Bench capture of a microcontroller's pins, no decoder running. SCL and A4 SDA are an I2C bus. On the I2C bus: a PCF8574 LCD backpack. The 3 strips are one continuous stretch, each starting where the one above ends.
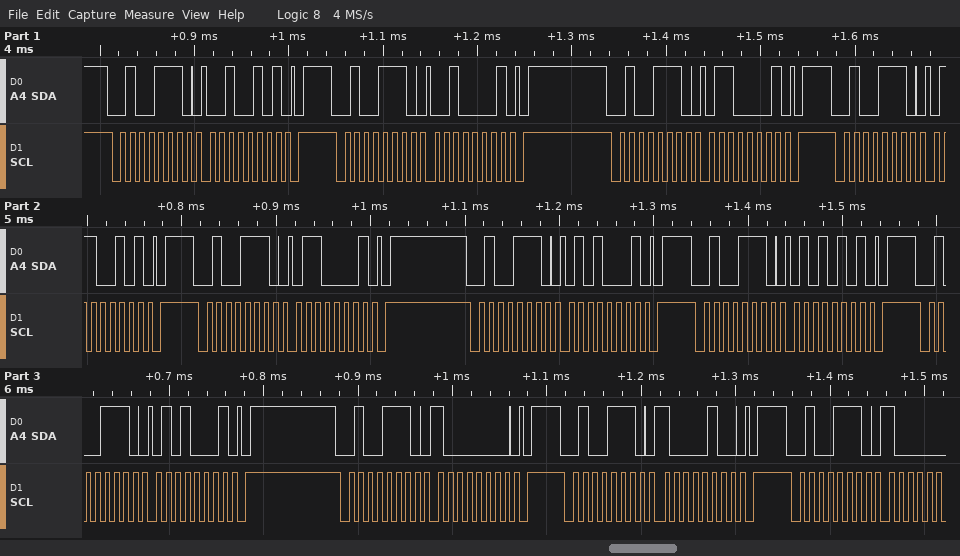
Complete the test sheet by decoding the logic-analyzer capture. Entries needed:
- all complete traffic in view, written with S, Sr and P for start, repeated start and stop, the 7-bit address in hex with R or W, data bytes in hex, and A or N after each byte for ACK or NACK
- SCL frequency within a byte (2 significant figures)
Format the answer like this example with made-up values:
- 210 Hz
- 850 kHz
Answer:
- S 27W A 25 A P S 27W A 21 A P S 27W A 61 A P S 27W A 65 A P S 27W A 61 A P S 27W A 51 A P S 27W A 55 A P S 27W A 51 A P S 27W A 80 A P S 27W A 84 A P S 27W A
- 100 kHz
